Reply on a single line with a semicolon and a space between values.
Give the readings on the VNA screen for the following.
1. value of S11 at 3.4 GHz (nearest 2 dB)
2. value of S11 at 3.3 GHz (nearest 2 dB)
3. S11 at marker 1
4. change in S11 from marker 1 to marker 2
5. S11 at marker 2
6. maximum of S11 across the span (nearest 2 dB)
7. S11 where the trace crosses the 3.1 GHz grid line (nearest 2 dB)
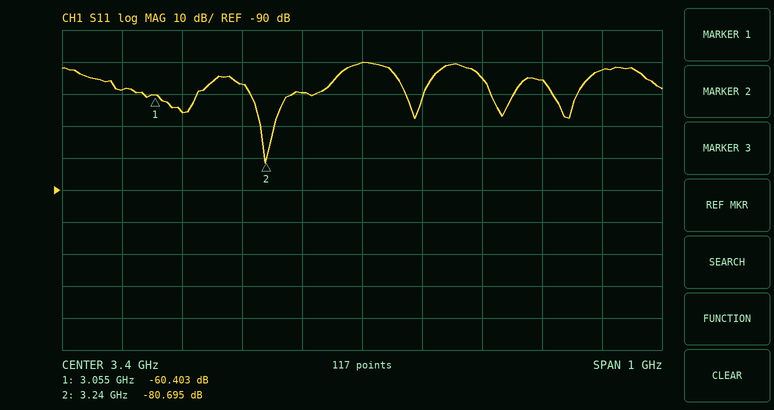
-50 dB; -60 dB; -60.403 dB; -20.292 dB; -80.695 dB; -50 dB; -66 dB
